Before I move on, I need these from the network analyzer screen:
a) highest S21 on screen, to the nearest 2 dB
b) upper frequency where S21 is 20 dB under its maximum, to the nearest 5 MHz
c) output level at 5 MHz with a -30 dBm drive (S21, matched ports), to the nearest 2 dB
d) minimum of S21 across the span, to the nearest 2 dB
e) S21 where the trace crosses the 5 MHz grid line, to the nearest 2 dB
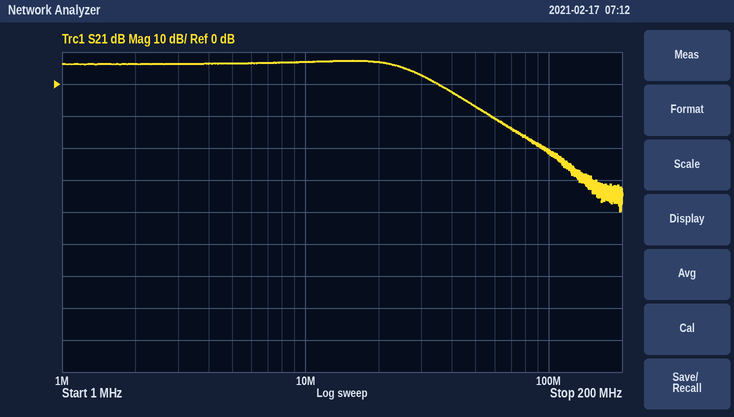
8 dB
65 MHz
-24 dBm
-40 dB
6 dB
